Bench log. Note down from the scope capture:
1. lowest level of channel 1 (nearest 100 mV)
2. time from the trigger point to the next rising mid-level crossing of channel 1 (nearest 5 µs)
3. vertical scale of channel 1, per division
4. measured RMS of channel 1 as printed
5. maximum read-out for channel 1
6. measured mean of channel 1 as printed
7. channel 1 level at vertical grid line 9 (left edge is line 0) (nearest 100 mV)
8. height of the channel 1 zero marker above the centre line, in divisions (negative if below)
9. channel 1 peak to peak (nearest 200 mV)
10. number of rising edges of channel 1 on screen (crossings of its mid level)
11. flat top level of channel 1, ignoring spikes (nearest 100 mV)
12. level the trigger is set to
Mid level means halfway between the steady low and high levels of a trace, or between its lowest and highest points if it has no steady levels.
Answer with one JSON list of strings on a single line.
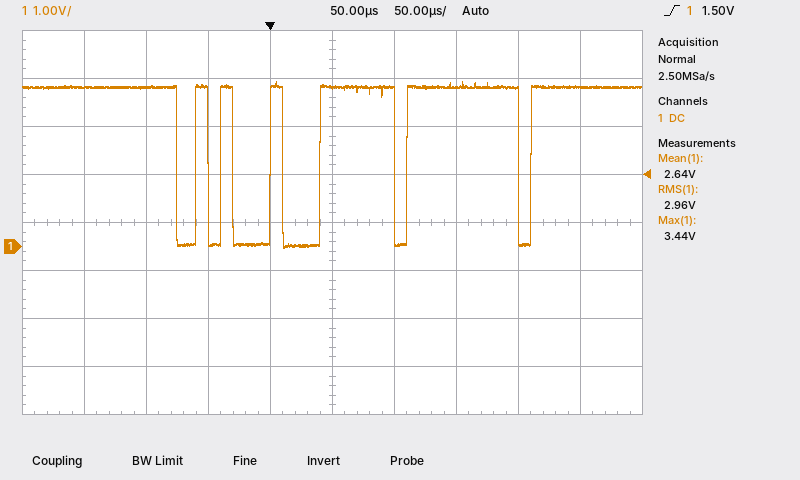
["0.0 V", "40 µs", "1 V", "2.96 V", "3.44 V", "2.64 V", "3.3 V", "-0.5 div", "3.4 V", "6", "3.3 V", "1.50 V"]
